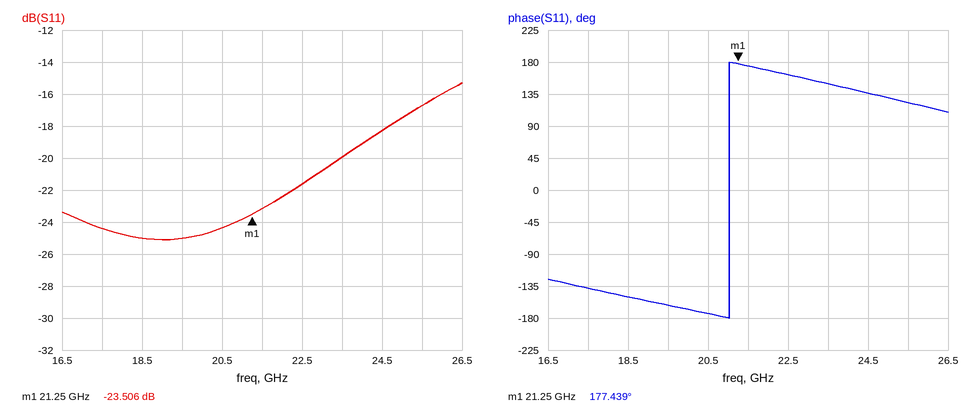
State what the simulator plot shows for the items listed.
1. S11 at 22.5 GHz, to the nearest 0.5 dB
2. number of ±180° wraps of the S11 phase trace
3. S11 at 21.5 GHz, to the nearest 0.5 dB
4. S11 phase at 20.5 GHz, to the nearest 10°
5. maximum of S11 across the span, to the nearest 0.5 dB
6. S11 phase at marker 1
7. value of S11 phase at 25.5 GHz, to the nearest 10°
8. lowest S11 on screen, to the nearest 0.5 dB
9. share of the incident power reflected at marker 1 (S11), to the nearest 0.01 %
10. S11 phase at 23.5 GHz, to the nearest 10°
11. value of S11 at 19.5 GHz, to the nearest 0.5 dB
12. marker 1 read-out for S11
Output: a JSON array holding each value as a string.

["-21.5 dB", "1", "-23.0 dB", "-170°", "-15.5 dB", "177.439°", "120°", "-25.0 dB", "0.45 %", "150°", "-25.0 dB", "-23.506 dB"]
